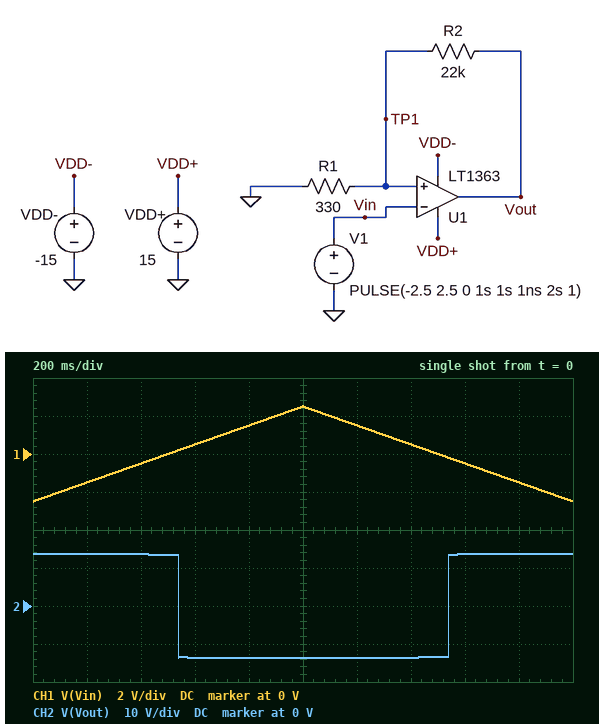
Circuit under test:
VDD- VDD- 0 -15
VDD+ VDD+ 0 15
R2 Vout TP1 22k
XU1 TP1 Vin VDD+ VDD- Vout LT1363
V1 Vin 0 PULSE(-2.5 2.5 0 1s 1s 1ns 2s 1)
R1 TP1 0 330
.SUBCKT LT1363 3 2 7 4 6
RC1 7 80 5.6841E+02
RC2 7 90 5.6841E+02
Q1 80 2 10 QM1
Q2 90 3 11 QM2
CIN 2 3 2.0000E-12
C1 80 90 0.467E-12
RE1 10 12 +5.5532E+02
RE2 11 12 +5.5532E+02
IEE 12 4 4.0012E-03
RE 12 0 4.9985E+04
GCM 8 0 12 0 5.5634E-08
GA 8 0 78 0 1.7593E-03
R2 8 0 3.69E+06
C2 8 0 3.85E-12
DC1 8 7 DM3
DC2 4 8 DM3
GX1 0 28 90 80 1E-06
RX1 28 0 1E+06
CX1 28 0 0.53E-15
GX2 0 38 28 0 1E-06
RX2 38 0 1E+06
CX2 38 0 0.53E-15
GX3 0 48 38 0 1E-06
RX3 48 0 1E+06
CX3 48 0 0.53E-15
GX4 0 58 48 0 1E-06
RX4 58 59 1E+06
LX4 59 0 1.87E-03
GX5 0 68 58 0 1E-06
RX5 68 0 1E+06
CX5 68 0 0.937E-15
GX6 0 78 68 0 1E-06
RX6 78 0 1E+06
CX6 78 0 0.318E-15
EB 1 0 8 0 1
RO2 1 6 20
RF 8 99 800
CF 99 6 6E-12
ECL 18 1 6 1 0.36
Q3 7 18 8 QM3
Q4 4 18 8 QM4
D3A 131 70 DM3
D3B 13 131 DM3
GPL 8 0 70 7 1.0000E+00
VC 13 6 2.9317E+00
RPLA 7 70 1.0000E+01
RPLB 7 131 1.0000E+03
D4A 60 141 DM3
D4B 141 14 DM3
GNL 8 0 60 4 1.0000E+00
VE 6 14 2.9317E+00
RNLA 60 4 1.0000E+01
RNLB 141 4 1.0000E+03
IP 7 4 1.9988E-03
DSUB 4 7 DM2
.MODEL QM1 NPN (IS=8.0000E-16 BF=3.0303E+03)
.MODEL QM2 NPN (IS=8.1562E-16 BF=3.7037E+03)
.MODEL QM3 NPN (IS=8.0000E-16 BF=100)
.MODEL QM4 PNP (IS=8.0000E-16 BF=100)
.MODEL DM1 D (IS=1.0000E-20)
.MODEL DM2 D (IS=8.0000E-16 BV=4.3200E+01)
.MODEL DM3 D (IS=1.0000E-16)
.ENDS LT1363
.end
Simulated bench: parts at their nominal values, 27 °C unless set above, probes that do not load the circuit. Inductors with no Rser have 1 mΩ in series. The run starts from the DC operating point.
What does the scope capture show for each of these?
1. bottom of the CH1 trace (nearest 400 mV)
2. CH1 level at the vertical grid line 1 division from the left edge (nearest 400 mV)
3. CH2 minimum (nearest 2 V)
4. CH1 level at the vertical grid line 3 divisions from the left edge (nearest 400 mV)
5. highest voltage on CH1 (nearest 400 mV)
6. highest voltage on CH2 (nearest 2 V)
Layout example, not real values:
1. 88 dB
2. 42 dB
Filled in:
1. -2.4 V
2. -1.6 V
3. -14 V
4. 400 mV
5. 2.4 V
6. 14 V
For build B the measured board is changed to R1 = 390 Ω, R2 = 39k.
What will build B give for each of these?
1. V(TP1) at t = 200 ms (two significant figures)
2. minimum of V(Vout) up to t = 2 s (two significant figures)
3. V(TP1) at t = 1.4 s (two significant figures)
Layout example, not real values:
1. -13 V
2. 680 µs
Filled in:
1. 130 mV
2. -14 V
3. -130 mV
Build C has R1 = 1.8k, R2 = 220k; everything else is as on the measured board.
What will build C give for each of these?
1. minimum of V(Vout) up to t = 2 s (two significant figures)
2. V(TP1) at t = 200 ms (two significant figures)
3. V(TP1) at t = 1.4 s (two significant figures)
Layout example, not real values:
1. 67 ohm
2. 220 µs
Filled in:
1. -14 V
2. 110 mV
3. -110 mV
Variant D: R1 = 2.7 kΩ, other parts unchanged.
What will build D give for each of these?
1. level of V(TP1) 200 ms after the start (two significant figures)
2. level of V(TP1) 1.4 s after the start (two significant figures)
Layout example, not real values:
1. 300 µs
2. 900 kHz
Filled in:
1. 1.5 V
2. -1.5 V
